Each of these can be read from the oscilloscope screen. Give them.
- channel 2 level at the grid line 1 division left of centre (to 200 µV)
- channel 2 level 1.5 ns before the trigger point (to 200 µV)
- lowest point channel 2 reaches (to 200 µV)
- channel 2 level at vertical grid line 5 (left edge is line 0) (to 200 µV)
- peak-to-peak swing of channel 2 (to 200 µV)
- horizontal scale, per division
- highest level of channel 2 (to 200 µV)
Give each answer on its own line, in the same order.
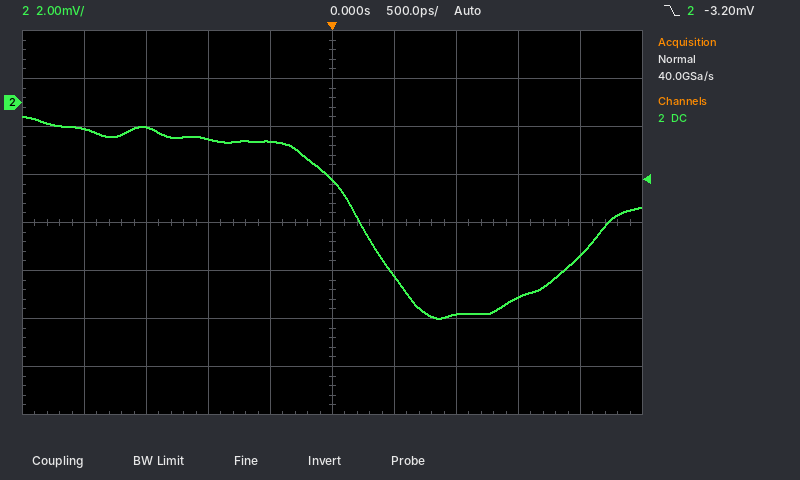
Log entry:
-1.6 mV
-1.0 mV
-9.0 mV
-3.2 mV
8.4 mV
500 ps
-600 µV
